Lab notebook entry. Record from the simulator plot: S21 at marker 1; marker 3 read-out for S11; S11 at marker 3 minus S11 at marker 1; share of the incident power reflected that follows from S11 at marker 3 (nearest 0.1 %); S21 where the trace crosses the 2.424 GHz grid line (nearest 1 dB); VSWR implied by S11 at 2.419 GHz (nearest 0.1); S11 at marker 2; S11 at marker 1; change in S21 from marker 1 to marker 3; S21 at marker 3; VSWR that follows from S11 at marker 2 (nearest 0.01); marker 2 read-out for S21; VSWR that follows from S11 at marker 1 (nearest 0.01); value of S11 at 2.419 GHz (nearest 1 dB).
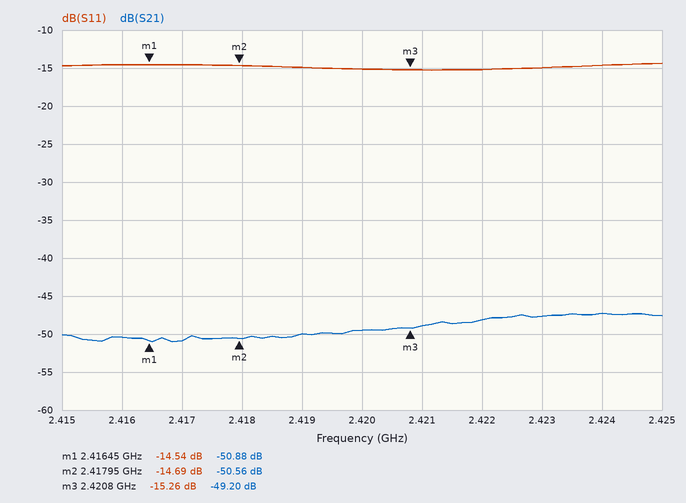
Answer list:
-50.88 dB
-15.26 dB
-0.72 dB
3.0 %
-47 dB
1.4
-14.69 dB
-14.54 dB
1.68 dB
-49.20 dB
1.45
-50.56 dB
1.46
-15 dB
